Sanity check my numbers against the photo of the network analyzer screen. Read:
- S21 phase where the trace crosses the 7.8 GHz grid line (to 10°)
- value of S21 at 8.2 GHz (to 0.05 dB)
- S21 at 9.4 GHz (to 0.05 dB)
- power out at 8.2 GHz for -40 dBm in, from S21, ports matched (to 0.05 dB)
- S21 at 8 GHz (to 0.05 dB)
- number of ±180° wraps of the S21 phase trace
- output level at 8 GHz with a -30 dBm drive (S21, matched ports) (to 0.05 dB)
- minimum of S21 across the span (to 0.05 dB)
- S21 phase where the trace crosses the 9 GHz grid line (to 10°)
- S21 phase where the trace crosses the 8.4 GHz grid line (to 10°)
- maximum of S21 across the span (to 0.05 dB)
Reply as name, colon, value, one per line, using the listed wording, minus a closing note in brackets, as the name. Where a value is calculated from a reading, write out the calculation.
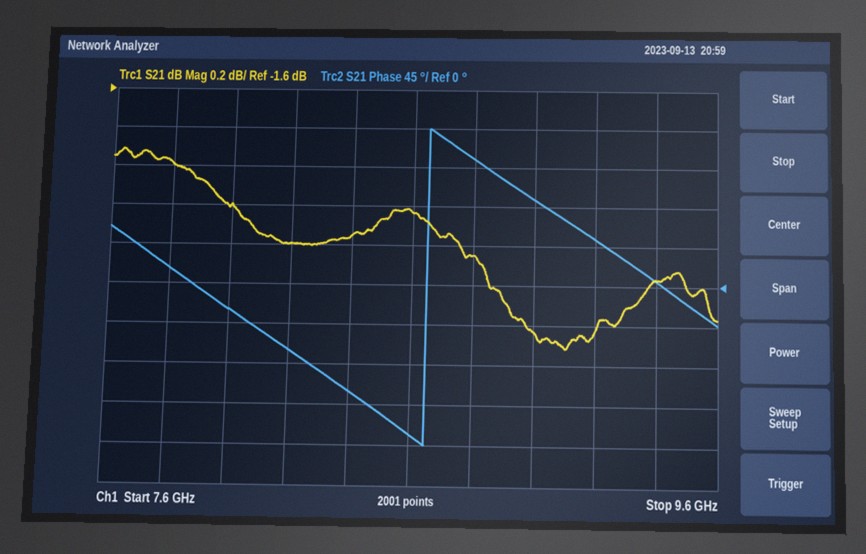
S21 phase where the trace crosses the 7.8 GHz grid line: 20°
value of S21 at 8.2 GHz: -2.40 dB
S21 at 9.4 GHz: -2.55 dB
power out at 8.2 GHz for -40 dBm in, from S21, ports matched: -40 dBm + (-2.40 dB) = -42.40 dBm
S21 at 8 GHz: -2.20 dB
number of ±180° wraps of the S21 phase trace: 1
output level at 8 GHz with a -30 dBm drive (S21, matched ports): -30 dBm + (-2.20 dB) = -32.20 dBm
minimum of S21 across the span: -2.90 dB
S21 phase where the trace crosses the 9 GHz grid line: 100°
S21 phase where the trace crosses the 8.4 GHz grid line: -120°
maximum of S21 across the span: -1.90 dB
